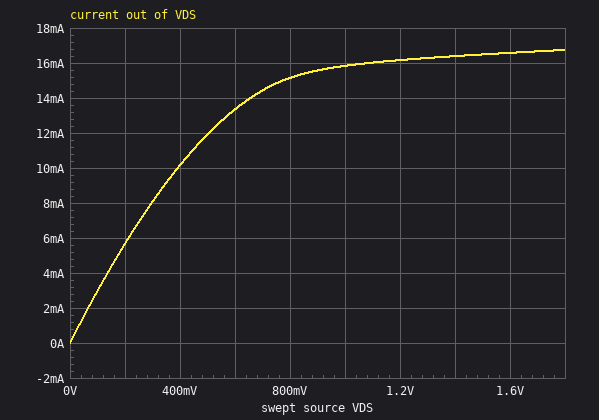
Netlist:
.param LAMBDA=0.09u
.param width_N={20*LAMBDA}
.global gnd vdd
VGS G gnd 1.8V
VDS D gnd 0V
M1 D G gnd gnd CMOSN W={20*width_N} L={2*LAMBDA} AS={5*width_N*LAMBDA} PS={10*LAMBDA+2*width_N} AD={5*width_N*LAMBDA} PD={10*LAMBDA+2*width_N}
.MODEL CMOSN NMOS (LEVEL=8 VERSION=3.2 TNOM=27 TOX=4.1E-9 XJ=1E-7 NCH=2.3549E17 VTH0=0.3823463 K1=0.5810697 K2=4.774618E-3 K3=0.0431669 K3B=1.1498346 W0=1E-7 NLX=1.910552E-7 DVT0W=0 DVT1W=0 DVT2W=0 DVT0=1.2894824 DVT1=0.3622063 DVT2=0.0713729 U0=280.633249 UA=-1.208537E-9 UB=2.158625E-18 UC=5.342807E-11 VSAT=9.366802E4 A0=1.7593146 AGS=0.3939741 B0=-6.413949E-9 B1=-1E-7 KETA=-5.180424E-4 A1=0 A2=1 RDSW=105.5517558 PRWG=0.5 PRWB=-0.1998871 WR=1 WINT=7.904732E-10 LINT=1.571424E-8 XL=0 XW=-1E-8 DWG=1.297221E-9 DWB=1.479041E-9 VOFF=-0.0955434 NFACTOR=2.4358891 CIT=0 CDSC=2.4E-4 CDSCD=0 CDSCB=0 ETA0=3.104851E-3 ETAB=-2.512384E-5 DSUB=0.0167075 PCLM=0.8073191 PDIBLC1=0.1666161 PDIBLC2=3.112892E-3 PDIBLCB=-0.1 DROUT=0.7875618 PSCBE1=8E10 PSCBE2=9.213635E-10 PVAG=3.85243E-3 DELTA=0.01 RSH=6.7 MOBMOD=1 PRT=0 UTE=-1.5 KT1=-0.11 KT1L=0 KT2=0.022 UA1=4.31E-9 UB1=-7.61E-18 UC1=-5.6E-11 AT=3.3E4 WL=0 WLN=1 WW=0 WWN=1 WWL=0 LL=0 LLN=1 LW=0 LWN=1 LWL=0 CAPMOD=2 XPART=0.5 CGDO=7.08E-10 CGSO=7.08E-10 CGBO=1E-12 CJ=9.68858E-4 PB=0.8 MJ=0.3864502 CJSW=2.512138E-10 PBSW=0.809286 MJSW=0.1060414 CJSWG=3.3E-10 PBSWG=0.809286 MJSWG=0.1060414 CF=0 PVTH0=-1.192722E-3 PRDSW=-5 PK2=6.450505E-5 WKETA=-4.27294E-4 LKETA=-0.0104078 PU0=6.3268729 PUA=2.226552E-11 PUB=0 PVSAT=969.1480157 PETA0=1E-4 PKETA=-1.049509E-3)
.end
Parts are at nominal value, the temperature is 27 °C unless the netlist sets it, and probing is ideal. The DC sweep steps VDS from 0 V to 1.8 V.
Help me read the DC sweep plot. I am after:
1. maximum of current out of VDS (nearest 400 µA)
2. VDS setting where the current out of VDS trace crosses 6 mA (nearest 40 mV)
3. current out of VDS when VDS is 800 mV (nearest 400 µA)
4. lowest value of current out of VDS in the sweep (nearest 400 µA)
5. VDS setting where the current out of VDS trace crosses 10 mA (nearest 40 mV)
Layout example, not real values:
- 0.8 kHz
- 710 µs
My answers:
- 16.8 mA
- 200 mV
- 15.2 mA
- 0 A
- 400 mV
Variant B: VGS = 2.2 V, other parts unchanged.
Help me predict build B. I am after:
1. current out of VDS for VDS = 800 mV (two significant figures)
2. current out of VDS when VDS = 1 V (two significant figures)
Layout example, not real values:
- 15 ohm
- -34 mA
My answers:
- 19 mA
- 21 mA
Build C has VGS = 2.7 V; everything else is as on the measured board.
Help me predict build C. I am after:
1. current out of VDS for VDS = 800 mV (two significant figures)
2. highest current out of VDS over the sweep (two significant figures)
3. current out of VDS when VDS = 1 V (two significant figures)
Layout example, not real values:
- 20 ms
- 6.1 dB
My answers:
- 21 mA
- 29 mA
- 24 mA
